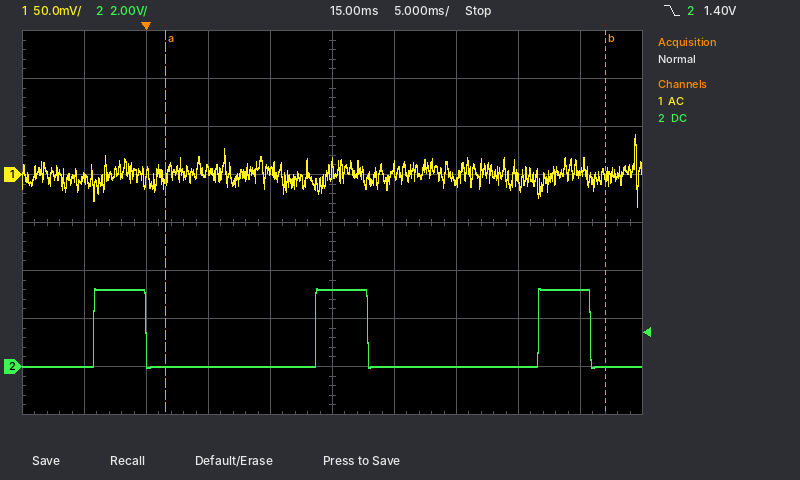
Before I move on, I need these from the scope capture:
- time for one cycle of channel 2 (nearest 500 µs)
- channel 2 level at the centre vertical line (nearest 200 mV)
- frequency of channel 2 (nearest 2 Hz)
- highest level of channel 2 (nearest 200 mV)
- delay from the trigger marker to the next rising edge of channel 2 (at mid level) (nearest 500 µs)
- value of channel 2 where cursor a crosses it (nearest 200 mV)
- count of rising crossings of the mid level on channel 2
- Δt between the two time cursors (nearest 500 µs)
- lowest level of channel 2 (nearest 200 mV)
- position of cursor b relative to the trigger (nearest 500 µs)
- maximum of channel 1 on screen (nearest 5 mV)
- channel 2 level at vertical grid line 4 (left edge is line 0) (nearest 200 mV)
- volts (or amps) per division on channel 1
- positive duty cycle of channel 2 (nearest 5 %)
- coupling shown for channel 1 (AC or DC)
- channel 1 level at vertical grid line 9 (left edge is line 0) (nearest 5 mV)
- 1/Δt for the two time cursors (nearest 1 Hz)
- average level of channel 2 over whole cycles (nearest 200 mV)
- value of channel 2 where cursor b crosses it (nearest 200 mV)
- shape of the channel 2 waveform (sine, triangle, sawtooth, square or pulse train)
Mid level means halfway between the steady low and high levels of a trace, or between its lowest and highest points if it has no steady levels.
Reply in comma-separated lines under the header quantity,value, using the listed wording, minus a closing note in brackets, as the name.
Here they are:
quantity,value
time for one cycle of channel 2,18.0 ms
channel 2 level at the centre vertical line,3.2 V
frequency of channel 2,56 Hz
highest level of channel 2,3.2 V
delay from the trigger marker to the next rising edge of channel 2 (at mid level),13.5 ms
value of channel 2 where cursor a crosses it,0.0 V
count of rising crossings of the mid level on channel 2,3
Δt between the two time cursors,35.5 ms
lowest level of channel 2,0.0 V
position of cursor b relative to the trigger,+37.0 ms
maximum of channel 1 on screen,40 mV
channel 2 level at vertical grid line 4 (left edge is line 0),0.0 V
volts (or amps) per division on channel 1,50 mV
positive duty cycle of channel 2,25 %
coupling shown for channel 1,AC
channel 1 level at vertical grid line 9 (left edge is line 0),0 mV
1/Δt for the two time cursors,28 Hz
average level of channel 2 over whole cycles,800 mV
value of channel 2 where cursor b crosses it,0.0 V
shape of the channel 2 waveform,pulse train
